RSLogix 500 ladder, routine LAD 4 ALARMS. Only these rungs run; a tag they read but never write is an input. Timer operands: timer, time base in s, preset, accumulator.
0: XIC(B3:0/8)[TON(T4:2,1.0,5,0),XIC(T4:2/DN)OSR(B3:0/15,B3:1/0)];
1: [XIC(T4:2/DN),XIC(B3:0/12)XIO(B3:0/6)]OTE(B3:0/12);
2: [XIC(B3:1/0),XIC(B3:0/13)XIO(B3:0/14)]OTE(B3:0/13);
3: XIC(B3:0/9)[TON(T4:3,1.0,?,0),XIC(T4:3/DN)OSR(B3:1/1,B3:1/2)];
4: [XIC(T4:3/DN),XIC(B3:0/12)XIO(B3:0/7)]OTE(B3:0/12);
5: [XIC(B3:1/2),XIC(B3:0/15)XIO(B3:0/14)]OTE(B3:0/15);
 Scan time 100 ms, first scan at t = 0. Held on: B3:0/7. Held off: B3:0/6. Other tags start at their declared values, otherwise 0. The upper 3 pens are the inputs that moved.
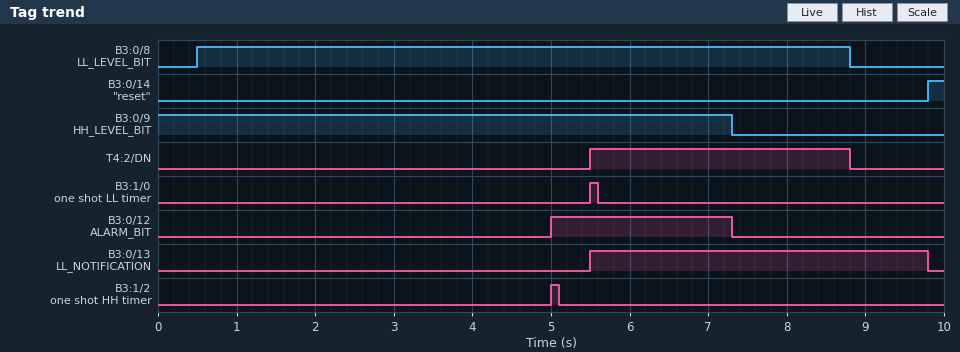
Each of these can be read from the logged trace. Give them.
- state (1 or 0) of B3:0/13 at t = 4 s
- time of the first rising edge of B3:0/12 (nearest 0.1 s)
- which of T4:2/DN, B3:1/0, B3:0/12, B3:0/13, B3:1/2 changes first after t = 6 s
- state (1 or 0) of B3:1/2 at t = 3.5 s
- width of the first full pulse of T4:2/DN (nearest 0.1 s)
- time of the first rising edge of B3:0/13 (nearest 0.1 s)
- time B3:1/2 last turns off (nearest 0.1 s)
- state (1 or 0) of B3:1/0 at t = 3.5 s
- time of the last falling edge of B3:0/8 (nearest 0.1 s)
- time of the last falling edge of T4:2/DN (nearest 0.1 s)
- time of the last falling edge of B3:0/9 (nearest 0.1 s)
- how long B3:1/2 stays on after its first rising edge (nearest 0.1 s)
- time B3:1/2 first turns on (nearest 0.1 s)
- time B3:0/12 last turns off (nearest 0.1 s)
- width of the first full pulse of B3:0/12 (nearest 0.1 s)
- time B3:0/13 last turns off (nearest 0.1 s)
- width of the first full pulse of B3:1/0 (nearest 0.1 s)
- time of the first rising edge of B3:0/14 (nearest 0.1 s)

0
5.0 s
B3:0/12
0
3.3 s
5.5 s
5.1 s
0
8.8 s
8.8 s
7.3 s
0.1 s
5.0 s
7.3 s
2.3 s
9.8 s
0.1 s
9.8 s
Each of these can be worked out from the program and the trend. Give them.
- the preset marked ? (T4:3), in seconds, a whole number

5 s
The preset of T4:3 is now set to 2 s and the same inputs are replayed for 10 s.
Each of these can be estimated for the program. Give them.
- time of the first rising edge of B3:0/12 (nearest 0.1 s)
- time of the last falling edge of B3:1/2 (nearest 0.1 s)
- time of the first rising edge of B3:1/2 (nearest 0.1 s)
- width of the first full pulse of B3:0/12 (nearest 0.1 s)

2.0 s
2.1 s
2.0 s
5.3 s
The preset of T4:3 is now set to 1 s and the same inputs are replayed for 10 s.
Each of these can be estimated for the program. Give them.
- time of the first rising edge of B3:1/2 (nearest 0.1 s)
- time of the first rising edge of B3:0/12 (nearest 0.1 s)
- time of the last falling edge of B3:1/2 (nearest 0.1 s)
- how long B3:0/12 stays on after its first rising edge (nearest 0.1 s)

1.0 s
1.0 s
1.1 s
6.3 s
